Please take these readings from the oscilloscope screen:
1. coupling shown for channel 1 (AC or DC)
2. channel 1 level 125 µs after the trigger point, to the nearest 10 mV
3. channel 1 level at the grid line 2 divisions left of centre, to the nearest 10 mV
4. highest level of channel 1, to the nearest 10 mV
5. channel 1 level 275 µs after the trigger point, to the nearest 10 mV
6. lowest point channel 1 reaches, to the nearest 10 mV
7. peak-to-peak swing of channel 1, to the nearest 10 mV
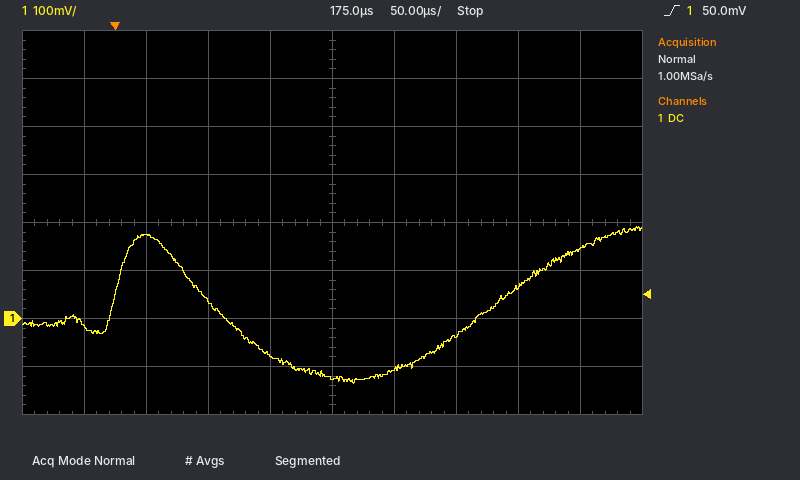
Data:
DC
-80 mV
40 mV
190 mV
-30 mV
-140 mV
330 mV
